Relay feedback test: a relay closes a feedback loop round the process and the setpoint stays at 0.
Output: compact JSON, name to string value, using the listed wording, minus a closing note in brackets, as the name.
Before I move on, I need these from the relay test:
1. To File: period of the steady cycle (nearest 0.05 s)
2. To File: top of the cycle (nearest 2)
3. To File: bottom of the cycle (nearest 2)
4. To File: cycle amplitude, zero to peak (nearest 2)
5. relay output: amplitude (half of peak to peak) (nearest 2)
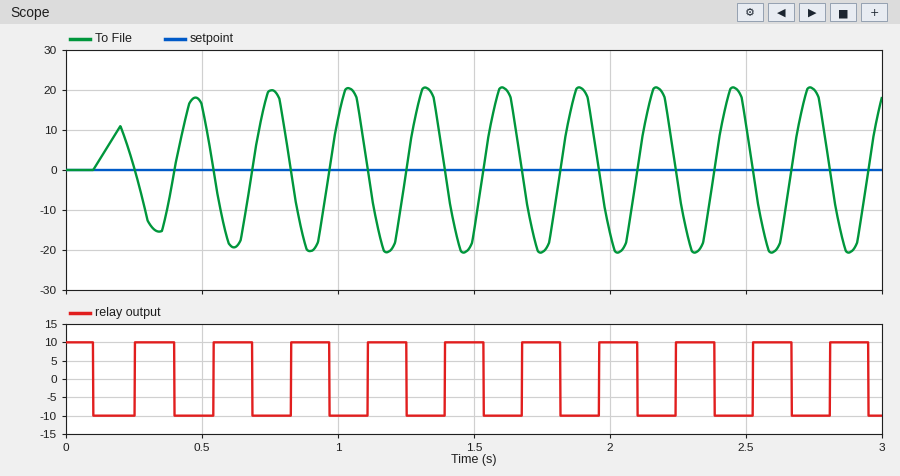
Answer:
{"To File: period of the steady cycle": "0.30 s", "To File: top of the cycle": "20", "To File: bottom of the cycle": "-20", "To File: cycle amplitude, zero to peak": "20", "relay output: amplitude (half of peak to peak)": "10"}
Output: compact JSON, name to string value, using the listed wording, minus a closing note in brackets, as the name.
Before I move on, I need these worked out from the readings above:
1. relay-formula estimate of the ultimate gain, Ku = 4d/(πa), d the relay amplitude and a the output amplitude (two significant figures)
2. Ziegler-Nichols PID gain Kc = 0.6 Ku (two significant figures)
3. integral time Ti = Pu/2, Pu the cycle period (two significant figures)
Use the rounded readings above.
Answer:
{"relay-formula estimate of the ultimate gain, Ku = 4d/(πa), d the relay amplitude and a the output amplitude": "0.64", "Ziegler-Nichols PID gain Kc = 0.6 Ku": "0.38", "integral time Ti = Pu/2, Pu the cycle period": "0.15 s"}
